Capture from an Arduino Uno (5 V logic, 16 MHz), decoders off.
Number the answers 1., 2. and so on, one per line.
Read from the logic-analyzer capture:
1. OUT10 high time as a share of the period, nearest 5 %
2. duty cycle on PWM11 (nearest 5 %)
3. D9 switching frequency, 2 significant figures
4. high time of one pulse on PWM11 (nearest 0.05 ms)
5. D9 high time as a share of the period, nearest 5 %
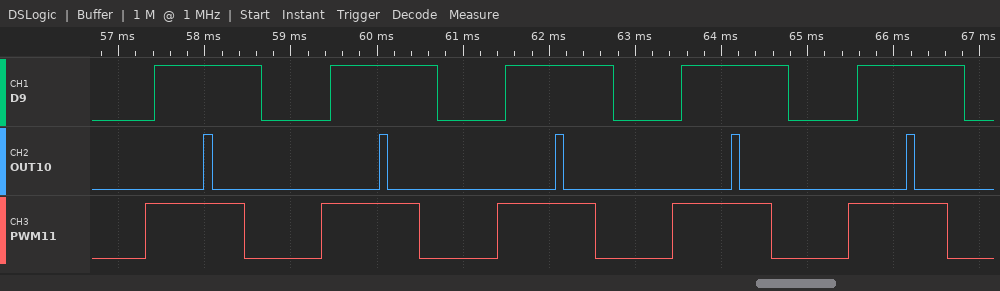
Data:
1. 5 %
2. 55 %
3. 490 Hz
4. 1.15 ms
5. 60 %
